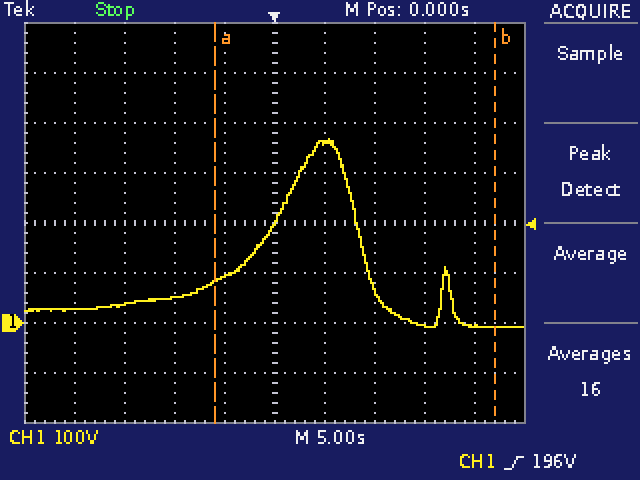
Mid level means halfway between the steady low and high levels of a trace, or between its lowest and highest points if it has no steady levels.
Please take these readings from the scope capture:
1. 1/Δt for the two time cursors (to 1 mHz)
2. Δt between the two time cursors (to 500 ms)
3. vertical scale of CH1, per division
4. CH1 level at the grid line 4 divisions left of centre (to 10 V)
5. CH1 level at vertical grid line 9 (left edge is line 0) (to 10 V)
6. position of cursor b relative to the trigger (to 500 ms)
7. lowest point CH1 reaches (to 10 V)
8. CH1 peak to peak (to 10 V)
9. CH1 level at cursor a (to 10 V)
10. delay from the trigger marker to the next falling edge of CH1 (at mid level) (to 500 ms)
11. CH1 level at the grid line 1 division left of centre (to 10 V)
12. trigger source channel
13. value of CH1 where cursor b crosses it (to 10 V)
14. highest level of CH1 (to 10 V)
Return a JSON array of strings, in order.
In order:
["36 mHz", "28.0 s", "100 V", "30 V", "-10 V", "+22.0 s", "-10 V", "380 V", "80 V", "8.5 s", "90 V", "CH1", "-10 V", "370 V"]
